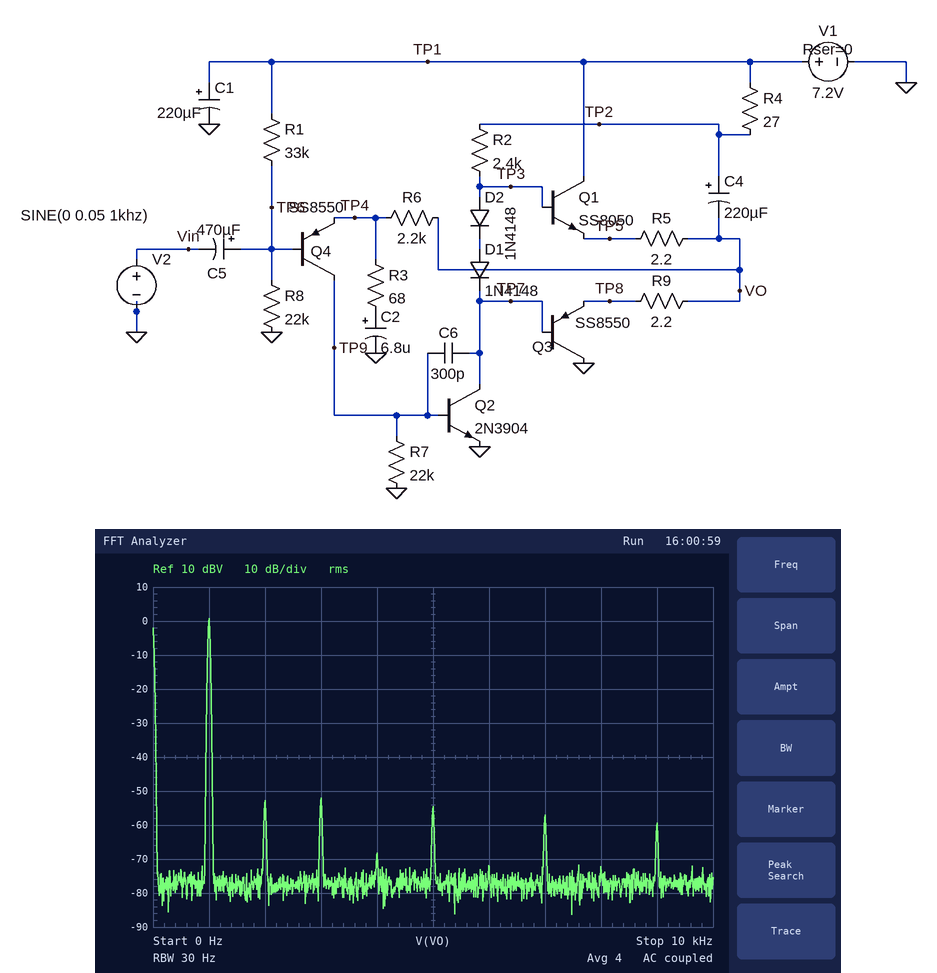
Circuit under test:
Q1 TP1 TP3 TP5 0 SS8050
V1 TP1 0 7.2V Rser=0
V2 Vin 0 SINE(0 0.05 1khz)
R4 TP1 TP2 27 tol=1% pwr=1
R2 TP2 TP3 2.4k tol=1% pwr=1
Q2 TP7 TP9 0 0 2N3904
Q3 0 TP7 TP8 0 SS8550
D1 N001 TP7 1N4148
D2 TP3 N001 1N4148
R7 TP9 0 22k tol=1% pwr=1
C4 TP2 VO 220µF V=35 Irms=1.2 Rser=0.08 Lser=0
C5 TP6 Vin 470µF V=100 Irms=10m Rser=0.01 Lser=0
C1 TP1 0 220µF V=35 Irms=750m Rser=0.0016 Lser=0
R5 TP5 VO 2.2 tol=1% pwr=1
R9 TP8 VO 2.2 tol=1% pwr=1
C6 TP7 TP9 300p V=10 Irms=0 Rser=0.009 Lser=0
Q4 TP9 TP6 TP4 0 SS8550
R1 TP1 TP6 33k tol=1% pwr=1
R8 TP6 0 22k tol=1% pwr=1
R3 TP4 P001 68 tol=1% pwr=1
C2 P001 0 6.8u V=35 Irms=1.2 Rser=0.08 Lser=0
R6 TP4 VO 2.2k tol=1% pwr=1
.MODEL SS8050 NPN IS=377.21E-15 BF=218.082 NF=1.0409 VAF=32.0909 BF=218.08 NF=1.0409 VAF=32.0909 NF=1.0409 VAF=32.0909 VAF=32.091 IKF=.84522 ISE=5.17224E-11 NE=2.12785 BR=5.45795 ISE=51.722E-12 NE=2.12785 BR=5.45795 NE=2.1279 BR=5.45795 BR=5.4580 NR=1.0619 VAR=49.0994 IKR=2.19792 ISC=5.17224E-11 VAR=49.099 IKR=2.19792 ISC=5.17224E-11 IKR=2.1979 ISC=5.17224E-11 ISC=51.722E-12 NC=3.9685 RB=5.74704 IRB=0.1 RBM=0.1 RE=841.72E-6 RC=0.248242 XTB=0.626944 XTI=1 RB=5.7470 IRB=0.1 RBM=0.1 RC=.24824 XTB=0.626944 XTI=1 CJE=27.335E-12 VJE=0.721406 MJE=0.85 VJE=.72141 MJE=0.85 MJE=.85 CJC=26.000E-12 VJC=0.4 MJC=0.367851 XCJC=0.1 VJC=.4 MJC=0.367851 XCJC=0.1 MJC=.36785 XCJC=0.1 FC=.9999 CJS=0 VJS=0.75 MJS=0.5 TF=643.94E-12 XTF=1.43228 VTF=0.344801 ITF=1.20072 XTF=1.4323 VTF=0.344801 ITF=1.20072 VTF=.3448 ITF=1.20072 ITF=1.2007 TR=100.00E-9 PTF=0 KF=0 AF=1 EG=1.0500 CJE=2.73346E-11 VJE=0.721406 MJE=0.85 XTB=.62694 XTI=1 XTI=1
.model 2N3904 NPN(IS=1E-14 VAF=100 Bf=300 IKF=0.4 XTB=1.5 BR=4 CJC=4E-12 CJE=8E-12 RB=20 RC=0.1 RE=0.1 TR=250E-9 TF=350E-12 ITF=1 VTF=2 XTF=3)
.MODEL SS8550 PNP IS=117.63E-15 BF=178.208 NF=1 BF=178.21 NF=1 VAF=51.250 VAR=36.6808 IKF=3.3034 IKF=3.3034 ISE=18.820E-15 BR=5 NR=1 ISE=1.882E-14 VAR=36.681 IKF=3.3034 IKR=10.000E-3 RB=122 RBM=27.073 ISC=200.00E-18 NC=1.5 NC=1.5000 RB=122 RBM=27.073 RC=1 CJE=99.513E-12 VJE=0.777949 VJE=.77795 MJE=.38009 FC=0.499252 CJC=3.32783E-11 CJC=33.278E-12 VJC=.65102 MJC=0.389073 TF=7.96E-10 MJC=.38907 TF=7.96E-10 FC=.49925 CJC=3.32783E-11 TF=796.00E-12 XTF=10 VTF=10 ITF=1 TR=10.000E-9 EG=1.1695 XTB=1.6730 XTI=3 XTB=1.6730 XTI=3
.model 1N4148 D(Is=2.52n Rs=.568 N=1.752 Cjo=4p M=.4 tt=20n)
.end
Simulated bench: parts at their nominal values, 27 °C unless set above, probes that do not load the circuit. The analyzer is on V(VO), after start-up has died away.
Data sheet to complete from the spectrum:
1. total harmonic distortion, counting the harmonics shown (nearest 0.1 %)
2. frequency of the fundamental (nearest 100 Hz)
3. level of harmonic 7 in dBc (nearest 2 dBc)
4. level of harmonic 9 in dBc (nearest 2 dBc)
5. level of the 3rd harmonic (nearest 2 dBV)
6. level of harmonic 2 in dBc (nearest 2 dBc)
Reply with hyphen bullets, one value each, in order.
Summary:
- 0.4 %
- 1.0 kHz
- -58 dBc
- -60 dBc
- -52 dBV
- -54 dBc
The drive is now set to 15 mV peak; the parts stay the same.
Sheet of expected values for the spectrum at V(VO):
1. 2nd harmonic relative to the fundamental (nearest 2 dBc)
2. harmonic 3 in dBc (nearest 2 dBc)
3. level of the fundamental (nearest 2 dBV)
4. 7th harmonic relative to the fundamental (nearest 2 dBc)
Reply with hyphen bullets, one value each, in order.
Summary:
- -58 dBc
- -48 dBc
- -10 dBV
- -60 dBc
